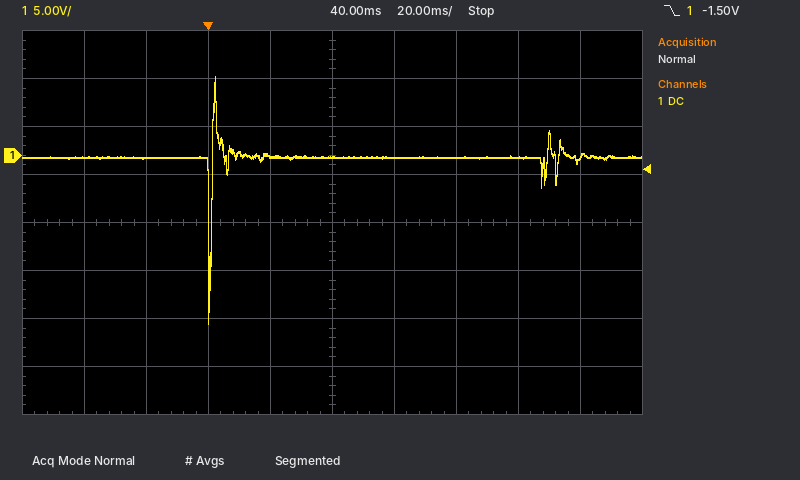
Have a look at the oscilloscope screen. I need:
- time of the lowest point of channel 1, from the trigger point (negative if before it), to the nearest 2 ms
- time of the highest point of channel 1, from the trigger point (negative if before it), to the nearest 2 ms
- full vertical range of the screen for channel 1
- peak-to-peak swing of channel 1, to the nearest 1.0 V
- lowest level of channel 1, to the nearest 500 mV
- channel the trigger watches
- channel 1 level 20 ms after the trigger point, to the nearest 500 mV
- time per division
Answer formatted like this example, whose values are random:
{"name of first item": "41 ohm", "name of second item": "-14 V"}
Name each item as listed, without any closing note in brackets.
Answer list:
{"time of the lowest point of channel 1, from the trigger point (negative if before it), to the nearest 2 ms": "0 ms", "time of the highest point of channel 1, from the trigger point (negative if before it), to the nearest 2 ms": "+2 ms", "full vertical range of the screen for channel 1": "40 V", "peak-to-peak swing of channel 1, to the nearest 1.0 V": "26.0 V", "lowest level of channel 1, to the nearest 500 mV": "-17.5 V", "channel the trigger watches": "channel 1", "channel 1 level 20 ms after the trigger point, to the nearest 500 mV": "0.0 V", "time per division": "20 ms"}
